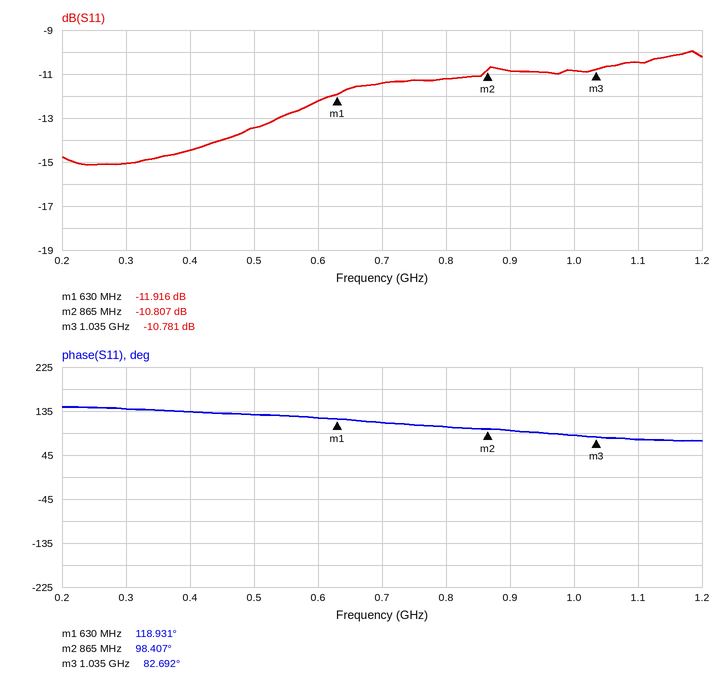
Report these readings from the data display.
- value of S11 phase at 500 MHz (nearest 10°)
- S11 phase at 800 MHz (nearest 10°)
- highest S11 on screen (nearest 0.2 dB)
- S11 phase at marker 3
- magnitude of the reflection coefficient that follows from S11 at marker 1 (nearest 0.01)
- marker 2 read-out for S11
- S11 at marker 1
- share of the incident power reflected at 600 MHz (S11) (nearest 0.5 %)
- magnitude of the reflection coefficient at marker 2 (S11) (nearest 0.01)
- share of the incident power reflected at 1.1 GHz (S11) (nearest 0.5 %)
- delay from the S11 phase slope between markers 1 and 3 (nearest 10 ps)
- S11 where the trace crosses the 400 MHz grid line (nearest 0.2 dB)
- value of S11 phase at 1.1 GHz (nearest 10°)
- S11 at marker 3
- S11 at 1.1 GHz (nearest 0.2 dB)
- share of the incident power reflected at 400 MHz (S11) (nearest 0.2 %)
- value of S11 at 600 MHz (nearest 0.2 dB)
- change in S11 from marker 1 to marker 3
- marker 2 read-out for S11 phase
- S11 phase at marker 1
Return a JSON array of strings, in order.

["130°", "100°", "-10.0 dB", "82.692°", "0.25", "-10.807 dB", "-11.916 dB", "6.0 %", "0.29", "9.0 %", "250 ps", "-14.4 dB", "80°", "-10.781 dB", "-10.4 dB", "3.6 %", "-12.2 dB", "1.135 dB", "98.407°", "118.931°"]
